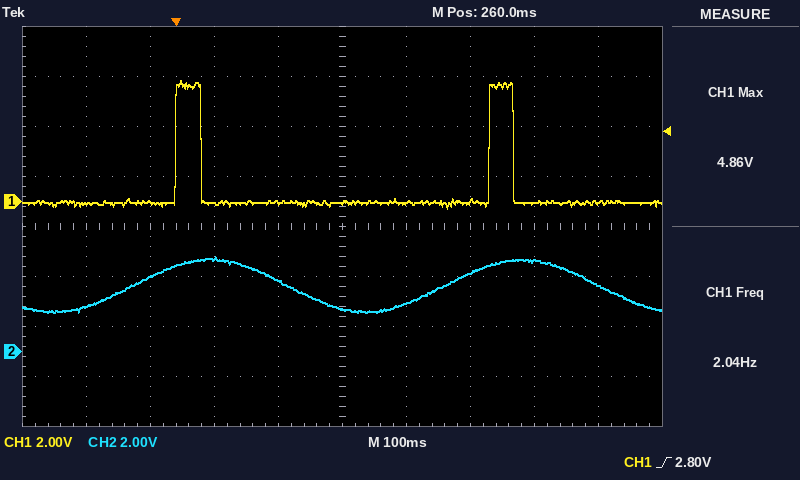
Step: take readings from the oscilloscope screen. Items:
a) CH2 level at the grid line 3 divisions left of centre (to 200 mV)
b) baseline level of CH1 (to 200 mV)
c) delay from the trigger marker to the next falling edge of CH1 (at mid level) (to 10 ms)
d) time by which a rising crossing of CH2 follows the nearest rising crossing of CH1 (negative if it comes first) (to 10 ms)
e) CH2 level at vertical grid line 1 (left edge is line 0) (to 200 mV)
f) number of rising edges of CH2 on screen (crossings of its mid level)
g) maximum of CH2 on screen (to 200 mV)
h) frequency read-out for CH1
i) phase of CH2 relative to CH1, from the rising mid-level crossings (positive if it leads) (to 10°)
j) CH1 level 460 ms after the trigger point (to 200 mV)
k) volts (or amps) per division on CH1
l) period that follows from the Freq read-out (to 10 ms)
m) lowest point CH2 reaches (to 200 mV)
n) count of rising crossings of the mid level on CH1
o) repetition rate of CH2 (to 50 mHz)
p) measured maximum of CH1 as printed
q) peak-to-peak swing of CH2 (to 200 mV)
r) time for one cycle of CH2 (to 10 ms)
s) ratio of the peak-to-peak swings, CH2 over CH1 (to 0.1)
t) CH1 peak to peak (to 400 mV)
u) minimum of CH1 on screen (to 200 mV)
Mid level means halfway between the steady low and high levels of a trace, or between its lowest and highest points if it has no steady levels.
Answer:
3.0 V
0.0 V
40 ms
-70 ms
1.8 V
2
3.8 V
2.04 Hz
+50°
0.0 V
2 V
490 ms
1.6 V
2
2.05 Hz
4.86 V
2.2 V
490 ms
0.4
5.2 V
-200 mV
